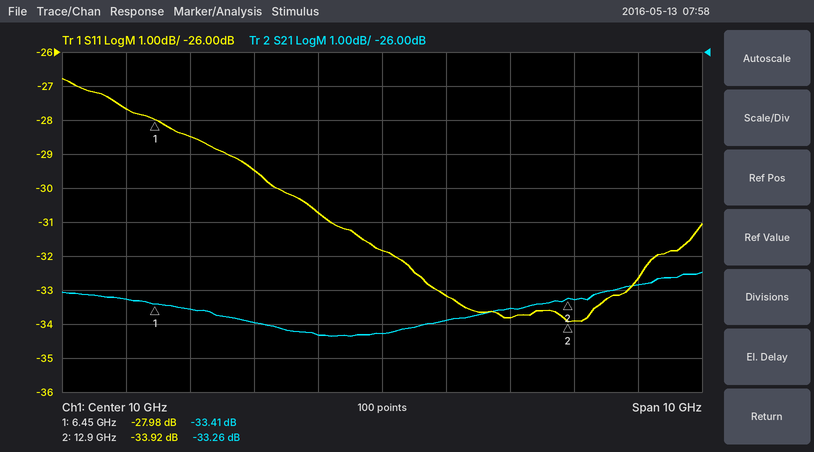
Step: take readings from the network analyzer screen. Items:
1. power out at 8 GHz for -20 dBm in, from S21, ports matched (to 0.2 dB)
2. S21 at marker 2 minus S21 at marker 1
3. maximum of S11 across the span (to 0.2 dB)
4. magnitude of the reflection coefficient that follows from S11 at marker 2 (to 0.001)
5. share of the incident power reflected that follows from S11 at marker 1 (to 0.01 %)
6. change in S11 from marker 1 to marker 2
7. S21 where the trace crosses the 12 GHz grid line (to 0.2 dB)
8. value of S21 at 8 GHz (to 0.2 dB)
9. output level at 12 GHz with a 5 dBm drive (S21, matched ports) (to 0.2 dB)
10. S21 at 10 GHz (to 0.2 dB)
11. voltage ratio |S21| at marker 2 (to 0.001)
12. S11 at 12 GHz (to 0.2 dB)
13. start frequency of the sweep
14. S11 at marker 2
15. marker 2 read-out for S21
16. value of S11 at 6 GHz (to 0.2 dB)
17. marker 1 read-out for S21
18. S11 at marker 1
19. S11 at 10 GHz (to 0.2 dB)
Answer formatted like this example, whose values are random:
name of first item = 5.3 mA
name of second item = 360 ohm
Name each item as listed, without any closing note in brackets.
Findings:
power out at 8 GHz for -20 dBm in, from S21, ports matched = -54.0 dBm
S21 at marker 2 minus S21 at marker 1 = 0.15 dB
maximum of S11 across the span = -26.8 dB
magnitude of the reflection coefficient that follows from S11 at marker 2 = 0.020
share of the incident power reflected that follows from S11 at marker 1 = 0.16 %
change in S11 from marker 1 to marker 2 = -5.94 dB
S21 where the trace crosses the 12 GHz grid line = -33.6 dB
value of S21 at 8 GHz = -34.0 dB
output level at 12 GHz with a 5 dBm drive (S21, matched ports) = -28.6 dBm
S21 at 10 GHz = -34.2 dB
voltage ratio |S21| at marker 2 = 0.022
S11 at 12 GHz = -33.8 dB
start frequency of the sweep = 5 GHz
S11 at marker 2 = -33.92 dB
marker 2 read-out for S21 = -33.26 dB
value of S11 at 6 GHz = -27.6 dB
marker 1 read-out for S21 = -33.41 dB
S11 at marker 1 = -27.98 dB
S11 at 10 GHz = -31.8 dB
